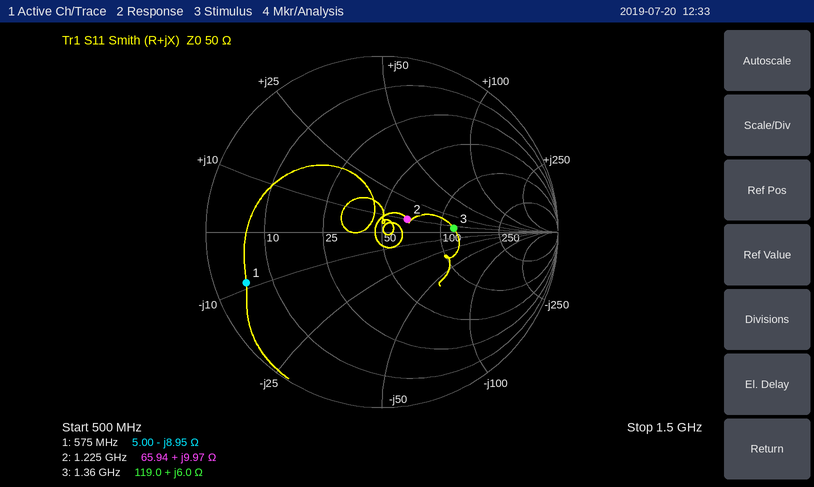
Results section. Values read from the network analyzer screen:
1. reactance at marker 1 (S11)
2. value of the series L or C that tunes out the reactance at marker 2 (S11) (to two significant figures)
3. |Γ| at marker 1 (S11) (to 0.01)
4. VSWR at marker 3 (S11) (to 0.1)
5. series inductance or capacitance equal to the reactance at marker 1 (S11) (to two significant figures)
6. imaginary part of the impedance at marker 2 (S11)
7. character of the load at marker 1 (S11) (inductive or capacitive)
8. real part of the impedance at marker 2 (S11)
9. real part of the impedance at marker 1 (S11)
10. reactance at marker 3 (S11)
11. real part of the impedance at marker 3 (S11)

-8.95 Ω
13 pF
0.82
2.4
31 pF
+9.97 Ω
capacitive
65.94 Ω
5.00 Ω
+6.0 Ω
119.0 Ω
